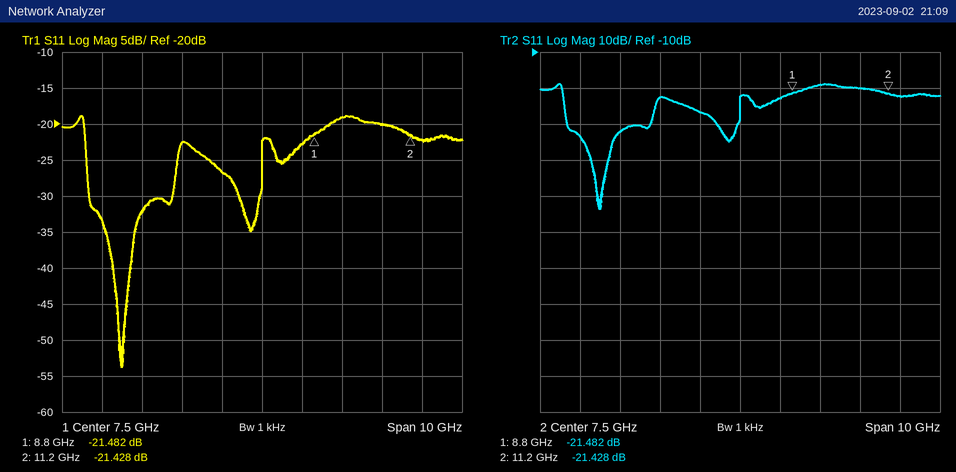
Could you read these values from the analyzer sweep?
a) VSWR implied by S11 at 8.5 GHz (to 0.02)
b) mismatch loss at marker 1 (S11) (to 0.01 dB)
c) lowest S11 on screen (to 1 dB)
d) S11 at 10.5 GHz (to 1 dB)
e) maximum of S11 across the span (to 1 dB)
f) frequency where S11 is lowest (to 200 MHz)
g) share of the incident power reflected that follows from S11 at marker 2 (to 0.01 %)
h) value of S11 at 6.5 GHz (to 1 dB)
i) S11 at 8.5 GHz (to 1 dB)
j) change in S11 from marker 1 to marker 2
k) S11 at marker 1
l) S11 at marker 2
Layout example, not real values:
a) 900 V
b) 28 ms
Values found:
a) 1.16
b) 0.03 dB
c) -54 dB
d) -20 dB
e) -19 dB
f) 4.0 GHz
g) 0.72 %
h) -27 dB
i) -23 dB
j) 0.054 dB
k) -21.482 dB
l) -21.428 dB
